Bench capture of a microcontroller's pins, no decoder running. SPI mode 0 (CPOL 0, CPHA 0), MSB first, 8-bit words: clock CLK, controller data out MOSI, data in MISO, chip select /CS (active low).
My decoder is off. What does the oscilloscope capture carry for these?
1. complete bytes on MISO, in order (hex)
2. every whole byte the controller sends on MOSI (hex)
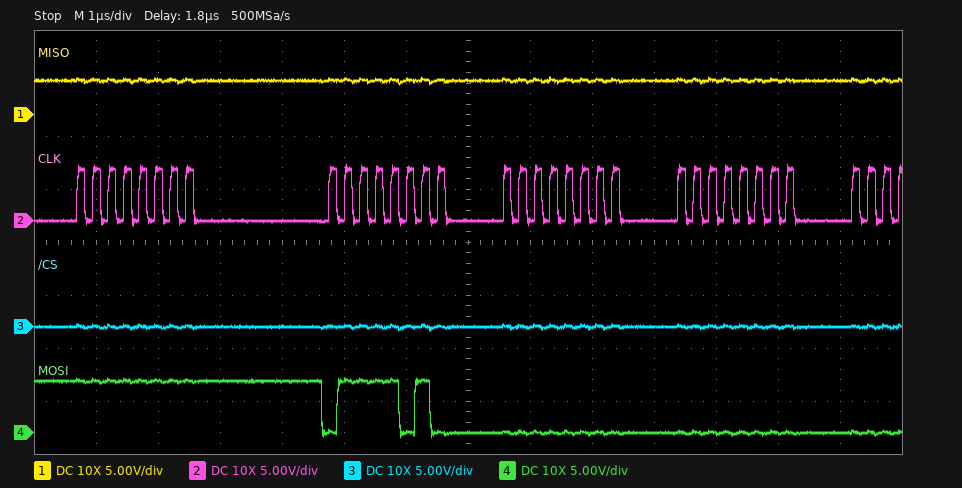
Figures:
FF FF FF FF
FF 7A 00 00
